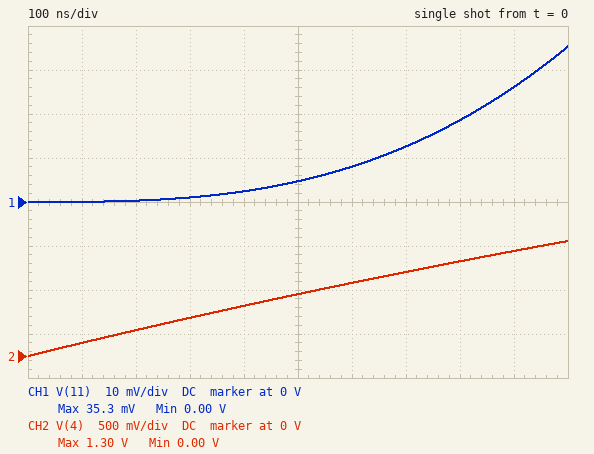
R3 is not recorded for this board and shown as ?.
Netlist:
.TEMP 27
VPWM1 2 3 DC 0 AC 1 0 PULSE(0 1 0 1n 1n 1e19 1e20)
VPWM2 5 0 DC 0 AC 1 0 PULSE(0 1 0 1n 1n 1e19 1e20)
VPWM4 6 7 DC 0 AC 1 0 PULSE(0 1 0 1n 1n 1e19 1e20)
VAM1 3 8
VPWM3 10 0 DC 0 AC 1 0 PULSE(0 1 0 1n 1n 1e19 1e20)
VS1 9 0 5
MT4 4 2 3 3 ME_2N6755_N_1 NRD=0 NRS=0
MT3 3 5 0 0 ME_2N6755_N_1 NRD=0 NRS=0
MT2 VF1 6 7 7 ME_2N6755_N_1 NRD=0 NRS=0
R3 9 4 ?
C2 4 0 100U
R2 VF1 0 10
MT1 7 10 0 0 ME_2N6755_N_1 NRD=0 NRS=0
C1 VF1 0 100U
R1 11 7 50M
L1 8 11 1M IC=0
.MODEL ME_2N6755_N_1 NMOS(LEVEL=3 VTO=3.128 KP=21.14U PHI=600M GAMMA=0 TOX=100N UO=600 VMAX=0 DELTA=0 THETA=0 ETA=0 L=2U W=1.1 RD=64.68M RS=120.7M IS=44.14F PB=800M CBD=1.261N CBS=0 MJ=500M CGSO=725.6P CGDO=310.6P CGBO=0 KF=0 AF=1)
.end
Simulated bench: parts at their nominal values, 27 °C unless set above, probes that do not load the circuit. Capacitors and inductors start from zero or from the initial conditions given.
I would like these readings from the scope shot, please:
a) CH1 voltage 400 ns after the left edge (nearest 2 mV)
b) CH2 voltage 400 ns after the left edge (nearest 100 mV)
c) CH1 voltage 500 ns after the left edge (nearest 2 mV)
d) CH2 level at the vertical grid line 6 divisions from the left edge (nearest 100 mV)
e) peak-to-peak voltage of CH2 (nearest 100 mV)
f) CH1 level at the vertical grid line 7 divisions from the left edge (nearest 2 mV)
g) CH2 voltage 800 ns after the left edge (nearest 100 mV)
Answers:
2 mV
600 mV
4 mV
800 mV
1.3 V
12 mV
1.1 V
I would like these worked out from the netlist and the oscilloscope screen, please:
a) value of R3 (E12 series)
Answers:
0.033 Ω
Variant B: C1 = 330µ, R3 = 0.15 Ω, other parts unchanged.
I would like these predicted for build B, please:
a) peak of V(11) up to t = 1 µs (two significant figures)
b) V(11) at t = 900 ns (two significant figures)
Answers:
8.3 mV
6.1 mV
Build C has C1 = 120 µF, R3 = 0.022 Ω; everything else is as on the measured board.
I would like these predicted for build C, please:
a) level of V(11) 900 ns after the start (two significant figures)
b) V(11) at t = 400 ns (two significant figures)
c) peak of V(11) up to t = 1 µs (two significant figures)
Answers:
38 mV
3.6 mV
51 mV
